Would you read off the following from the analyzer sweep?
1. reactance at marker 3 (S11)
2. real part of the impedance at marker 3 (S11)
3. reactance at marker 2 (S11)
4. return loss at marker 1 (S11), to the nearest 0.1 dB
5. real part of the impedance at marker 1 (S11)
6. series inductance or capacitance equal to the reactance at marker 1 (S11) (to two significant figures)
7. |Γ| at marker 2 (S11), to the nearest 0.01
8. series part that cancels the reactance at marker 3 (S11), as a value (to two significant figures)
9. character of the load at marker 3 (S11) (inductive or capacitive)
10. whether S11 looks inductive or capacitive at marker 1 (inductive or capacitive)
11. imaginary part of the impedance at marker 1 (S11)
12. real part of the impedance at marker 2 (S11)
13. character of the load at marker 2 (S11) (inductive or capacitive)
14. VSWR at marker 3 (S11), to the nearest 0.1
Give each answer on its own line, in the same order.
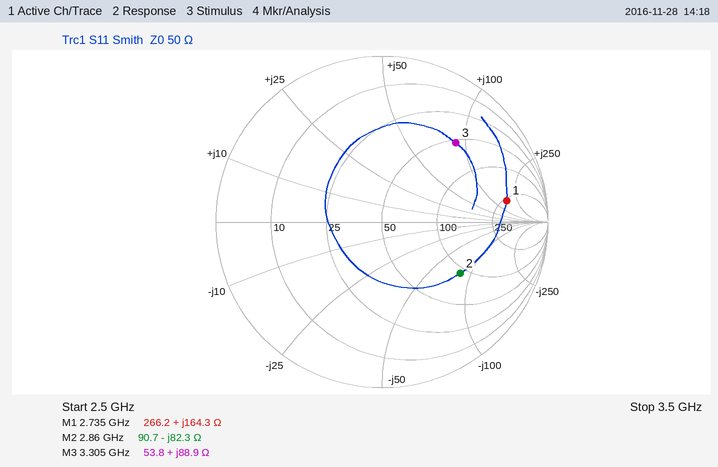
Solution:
+88.9 Ω
53.8 Ω
-82.3 Ω
2.4 dB
266.2 Ω
9.6 nH
0.56
540 fF
inductive
inductive
+164.3 Ω
90.7 Ω
capacitive
4.7
